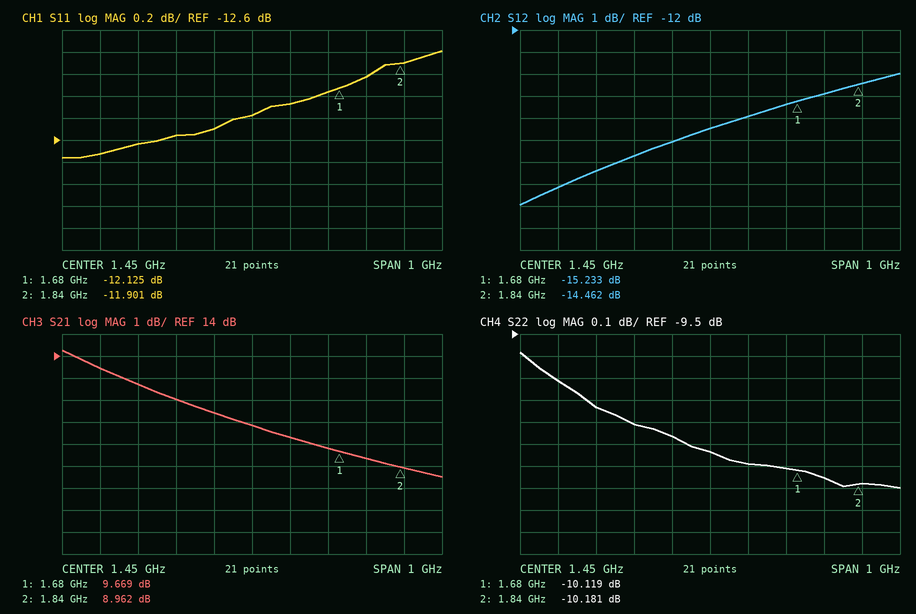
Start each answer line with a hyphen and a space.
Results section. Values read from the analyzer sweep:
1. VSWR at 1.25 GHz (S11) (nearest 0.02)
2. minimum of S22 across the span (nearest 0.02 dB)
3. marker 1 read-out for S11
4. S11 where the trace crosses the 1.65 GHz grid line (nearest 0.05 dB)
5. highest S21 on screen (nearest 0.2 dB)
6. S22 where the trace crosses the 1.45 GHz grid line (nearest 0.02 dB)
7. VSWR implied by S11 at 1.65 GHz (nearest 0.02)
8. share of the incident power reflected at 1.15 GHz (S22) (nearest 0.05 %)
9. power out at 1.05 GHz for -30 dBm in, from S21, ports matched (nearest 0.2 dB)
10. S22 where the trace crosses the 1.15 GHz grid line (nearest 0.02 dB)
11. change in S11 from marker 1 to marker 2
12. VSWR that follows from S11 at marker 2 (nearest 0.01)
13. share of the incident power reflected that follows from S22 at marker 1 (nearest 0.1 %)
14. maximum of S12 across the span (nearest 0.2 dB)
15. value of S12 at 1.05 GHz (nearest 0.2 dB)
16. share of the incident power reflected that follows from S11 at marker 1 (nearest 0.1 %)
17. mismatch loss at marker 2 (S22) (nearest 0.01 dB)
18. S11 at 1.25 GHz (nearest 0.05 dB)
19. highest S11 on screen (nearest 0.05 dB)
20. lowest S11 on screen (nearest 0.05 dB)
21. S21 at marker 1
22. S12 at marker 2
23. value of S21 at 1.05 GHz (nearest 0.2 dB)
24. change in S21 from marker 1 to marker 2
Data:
- 1.62
- -10.20 dB
- -12.125 dB
- -12.15 dB
- 14.2 dB
- -10.04 dB
- 1.66
- 10.40 %
- -16.6 dBm
- -9.84 dB
- 0.224 dB
- 1.68
- 9.7 %
- -14.0 dB
- -19.2 dB
- 6.1 %
- 0.44 dB
- -12.55 dB
- -11.80 dB
- -12.75 dB
- 9.669 dB
- -14.462 dB
- 13.4 dB
- -0.707 dB
